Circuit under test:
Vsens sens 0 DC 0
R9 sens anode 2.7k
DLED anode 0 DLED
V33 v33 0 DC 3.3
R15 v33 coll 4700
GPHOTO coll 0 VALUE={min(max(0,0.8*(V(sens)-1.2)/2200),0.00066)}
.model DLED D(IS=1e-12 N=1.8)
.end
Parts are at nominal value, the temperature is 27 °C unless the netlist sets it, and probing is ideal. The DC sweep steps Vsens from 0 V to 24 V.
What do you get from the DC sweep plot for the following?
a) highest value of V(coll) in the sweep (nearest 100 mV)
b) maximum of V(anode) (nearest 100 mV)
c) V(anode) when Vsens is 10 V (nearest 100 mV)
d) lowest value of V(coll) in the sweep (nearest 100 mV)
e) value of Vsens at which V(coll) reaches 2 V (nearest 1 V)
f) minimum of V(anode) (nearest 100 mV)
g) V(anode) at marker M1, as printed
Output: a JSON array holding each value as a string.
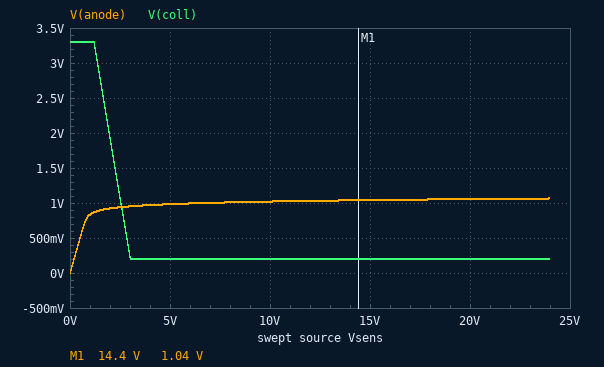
["3.3 V", "1.1 V", "1.0 V", "200 mV", "2 V", "0 V", "1.04 V"]
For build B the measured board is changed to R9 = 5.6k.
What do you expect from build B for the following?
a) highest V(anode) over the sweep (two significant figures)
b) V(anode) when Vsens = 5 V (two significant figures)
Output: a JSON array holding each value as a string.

["1.0 V", "950 mV"]
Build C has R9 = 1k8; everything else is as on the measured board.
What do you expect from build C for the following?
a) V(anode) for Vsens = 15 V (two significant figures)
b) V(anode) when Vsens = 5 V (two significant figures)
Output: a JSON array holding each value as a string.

["1.1 V", "1.0 V"]
